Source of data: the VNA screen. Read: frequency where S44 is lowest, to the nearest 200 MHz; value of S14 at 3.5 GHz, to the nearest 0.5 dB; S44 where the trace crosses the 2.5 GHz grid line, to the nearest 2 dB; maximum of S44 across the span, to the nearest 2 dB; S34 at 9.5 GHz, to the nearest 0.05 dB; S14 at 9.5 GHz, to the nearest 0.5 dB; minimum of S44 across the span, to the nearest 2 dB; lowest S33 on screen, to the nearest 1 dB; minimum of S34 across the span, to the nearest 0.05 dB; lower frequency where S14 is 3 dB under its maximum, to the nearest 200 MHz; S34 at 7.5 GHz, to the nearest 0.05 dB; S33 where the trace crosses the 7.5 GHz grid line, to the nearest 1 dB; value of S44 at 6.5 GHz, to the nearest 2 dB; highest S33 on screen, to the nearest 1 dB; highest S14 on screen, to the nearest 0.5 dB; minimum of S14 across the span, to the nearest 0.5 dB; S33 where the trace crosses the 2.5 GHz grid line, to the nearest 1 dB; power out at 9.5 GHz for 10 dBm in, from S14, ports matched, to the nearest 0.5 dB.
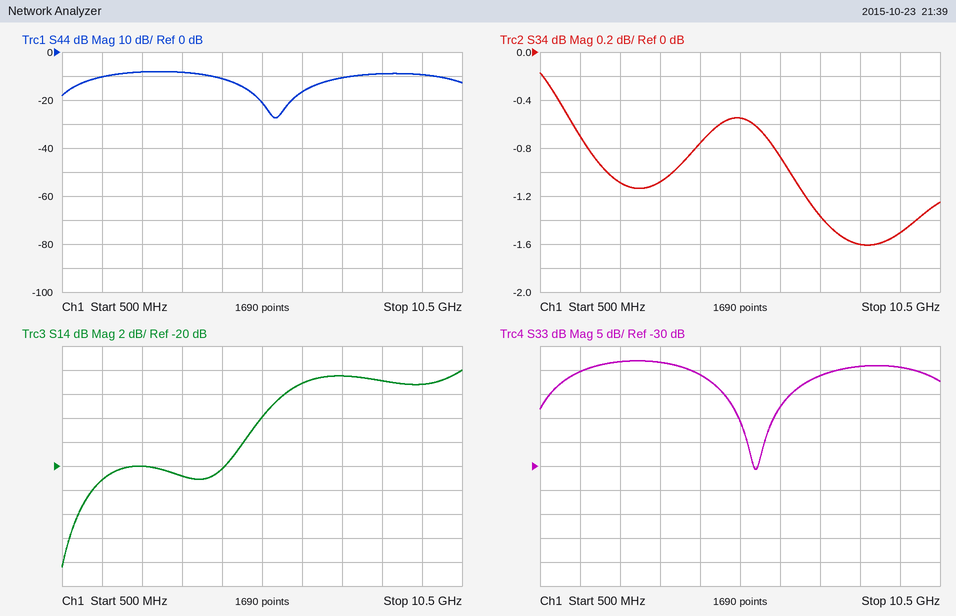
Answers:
5.8 GHz
-21.0 dB
-8 dB
-8 dB
-1.50 dB
-13.0 dB
-28 dB
-31 dB
-1.60 dB
5.8 GHz
-1.35 dB
-11 dB
-16 dB
-8 dB
-12.0 dB
-28.5 dB
-8 dB
-3.0 dBm
